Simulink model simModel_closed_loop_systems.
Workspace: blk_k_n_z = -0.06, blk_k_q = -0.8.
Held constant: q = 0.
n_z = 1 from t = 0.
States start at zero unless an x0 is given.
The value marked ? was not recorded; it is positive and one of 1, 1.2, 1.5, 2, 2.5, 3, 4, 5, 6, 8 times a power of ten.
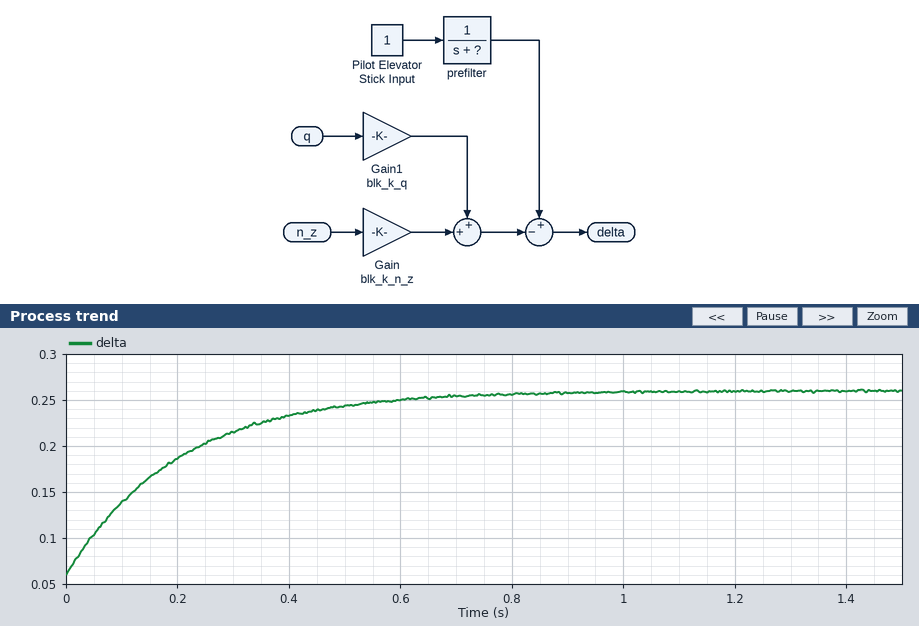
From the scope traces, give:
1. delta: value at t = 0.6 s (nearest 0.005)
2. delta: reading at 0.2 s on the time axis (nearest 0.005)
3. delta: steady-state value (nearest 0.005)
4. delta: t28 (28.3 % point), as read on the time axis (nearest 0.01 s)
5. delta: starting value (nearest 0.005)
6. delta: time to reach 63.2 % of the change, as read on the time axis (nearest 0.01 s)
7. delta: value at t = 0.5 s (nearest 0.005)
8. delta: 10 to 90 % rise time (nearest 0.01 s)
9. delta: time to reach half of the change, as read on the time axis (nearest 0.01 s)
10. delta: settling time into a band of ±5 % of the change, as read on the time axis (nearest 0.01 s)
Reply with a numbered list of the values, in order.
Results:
1. 0.250
2. 0.185
3. 0.260
4. 0.07 s
5. 0.060
6. 0.20 s
7. 0.245
8. 0.44 s
9. 0.14 s
10. 0.60 s
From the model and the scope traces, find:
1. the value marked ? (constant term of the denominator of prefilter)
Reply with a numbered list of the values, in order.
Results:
1. 5
